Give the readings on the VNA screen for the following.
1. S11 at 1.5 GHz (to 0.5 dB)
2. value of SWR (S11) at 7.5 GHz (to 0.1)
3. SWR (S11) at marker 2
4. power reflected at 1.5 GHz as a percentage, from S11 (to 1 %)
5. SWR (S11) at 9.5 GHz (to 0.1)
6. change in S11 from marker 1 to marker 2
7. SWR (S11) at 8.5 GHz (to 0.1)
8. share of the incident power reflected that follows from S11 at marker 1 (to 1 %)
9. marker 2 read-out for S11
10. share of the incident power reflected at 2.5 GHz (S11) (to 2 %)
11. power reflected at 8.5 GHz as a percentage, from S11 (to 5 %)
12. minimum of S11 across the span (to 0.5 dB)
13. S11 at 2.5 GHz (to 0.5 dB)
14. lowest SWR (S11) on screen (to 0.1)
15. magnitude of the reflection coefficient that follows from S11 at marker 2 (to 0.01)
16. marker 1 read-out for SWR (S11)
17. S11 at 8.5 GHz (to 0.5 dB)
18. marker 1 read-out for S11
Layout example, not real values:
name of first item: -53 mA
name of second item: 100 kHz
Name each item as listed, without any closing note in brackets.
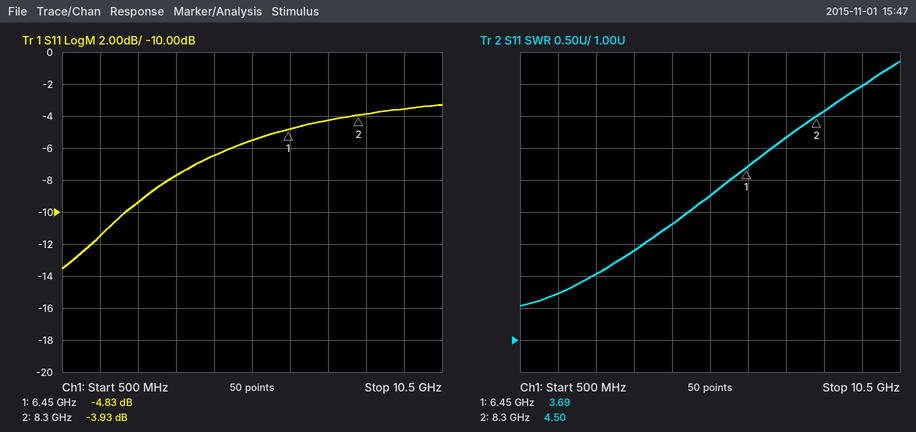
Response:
S11 at 1.5 GHz: -11.5 dB
value of SWR (S11) at 7.5 GHz: 4.2
SWR (S11) at marker 2: 4.50
power reflected at 1.5 GHz as a percentage, from S11: 7 %
SWR (S11) at 9.5 GHz: 5.0
change in S11 from marker 1 to marker 2: 0.90 dB
SWR (S11) at 8.5 GHz: 4.6
share of the incident power reflected that follows from S11 at marker 1: 33 %
marker 2 read-out for S11: -3.93 dB
share of the incident power reflected at 2.5 GHz (S11): 12 %
power reflected at 8.5 GHz as a percentage, from S11: 40 %
minimum of S11 across the span: -13.5 dB
S11 at 2.5 GHz: -9.5 dB
lowest SWR (S11) on screen: 1.5
magnitude of the reflection coefficient that follows from S11 at marker 2: 0.64
marker 1 read-out for SWR: 3.69
S11 at 8.5 GHz: -4.0 dB
marker 1 read-out for S11: -4.83 dB
